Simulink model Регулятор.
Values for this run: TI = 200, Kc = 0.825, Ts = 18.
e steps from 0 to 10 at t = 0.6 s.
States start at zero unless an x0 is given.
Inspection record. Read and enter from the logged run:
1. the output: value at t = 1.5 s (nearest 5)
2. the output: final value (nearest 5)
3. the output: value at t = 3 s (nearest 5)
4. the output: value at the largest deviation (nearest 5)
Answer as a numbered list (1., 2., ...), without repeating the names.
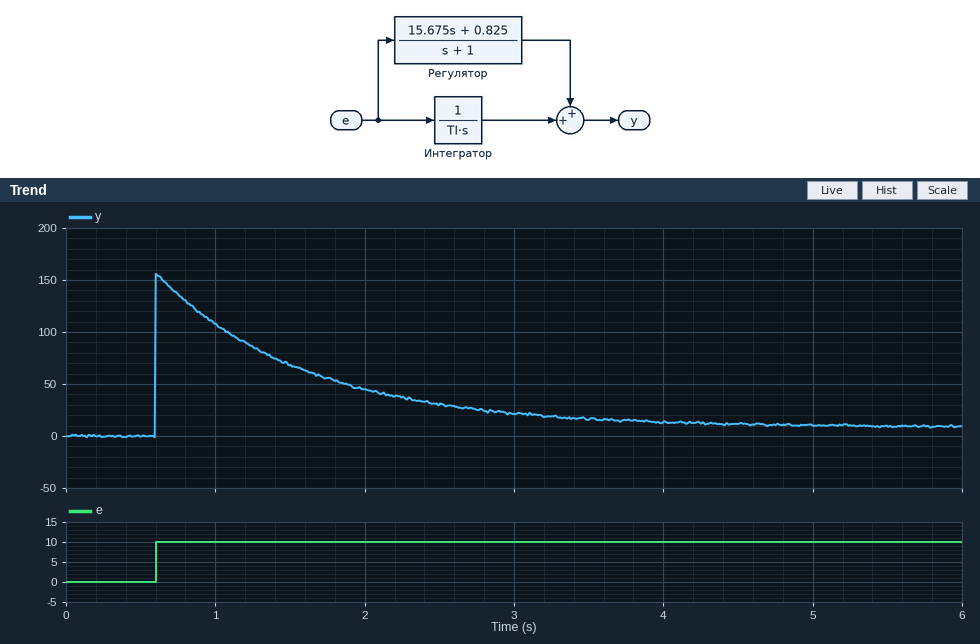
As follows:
1. 70
2. 10
3. 20
4. 155
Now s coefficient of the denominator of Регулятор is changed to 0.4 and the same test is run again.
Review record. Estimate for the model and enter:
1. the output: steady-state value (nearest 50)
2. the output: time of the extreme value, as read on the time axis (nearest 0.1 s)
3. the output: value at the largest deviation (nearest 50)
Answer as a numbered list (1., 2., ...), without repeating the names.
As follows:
1. 0
2. 0.6 s
3. 400
